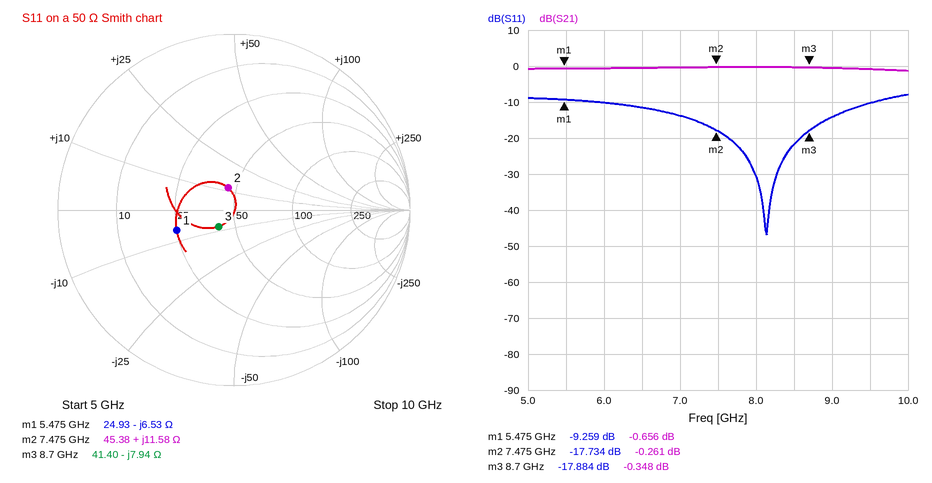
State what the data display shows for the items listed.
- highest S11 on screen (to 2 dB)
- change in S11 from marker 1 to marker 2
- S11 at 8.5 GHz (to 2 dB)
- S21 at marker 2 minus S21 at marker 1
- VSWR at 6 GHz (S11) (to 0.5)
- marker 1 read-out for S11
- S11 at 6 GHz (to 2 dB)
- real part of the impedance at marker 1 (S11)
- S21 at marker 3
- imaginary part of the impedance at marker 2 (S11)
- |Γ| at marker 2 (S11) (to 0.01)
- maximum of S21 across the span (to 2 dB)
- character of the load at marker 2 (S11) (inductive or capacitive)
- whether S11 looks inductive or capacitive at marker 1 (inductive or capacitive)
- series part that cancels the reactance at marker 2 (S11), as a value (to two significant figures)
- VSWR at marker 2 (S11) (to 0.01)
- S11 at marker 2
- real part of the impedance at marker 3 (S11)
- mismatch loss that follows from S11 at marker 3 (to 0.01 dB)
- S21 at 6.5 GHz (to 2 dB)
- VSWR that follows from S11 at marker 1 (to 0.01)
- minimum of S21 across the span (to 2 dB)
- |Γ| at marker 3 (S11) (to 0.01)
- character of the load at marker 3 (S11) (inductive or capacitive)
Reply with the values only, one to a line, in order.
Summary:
-8 dB
-8.475 dB
-22 dB
0.395 dB
2.0
-9.259 dB
-10 dB
24.93 Ω
-0.348 dB
+11.58 Ω
0.13
0 dB
inductive
capacitive
1.8 pF
1.30
-17.734 dB
41.40 Ω
0.07 dB
0 dB
2.05
-2 dB
0.13
capacitive
